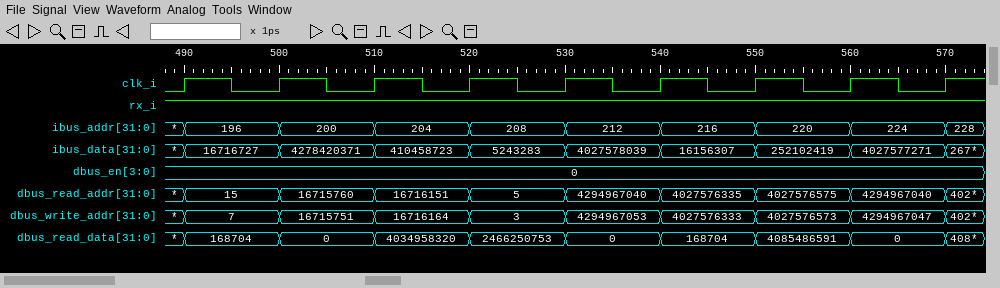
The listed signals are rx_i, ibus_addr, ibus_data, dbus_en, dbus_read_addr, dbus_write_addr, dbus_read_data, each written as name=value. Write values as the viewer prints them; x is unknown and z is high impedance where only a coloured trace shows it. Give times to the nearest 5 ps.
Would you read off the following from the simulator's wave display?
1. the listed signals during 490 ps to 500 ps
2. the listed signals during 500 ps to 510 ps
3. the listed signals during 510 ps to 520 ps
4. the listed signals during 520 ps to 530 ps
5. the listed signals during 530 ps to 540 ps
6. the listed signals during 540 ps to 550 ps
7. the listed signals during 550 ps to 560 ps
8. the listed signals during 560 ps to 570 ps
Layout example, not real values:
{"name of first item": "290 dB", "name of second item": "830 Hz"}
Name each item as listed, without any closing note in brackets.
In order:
{"the listed signals during 490 ps to 500 ps": "rx_i=1, ibus_addr=196, ibus_data=16716727, dbus_en=0, dbus_read_addr=15, dbus_write_addr=7, dbus_read_data=168704", "the listed signals during 500 ps to 510 ps": "rx_i=1, ibus_addr=200, ibus_data=4278420371, dbus_en=0, dbus_read_addr=16715760, dbus_write_addr=16715751, dbus_read_data=0", "the listed signals during 510 ps to 520 ps": "rx_i=1, ibus_addr=204, ibus_data=410458723, dbus_en=0, dbus_read_addr=16716151, dbus_write_addr=16716164, dbus_read_data=4034958320", "the listed signals during 520 ps to 530 ps": "rx_i=1, ibus_addr=208, ibus_data=5243283, dbus_en=0, dbus_read_addr=5, dbus_write_addr=3, dbus_read_data=2466250753", "the listed signals during 530 ps to 540 ps": "rx_i=1, ibus_addr=212, ibus_data=4027578039, dbus_en=0, dbus_read_addr=4294967040, dbus_write_addr=4294967053, dbus_read_data=0", "the listed signals during 540 ps to 550 ps": "rx_i=1, ibus_addr=216, ibus_data=16156307, dbus_en=0, dbus_read_addr=4027576335, dbus_write_addr=4027576333, dbus_read_data=168704", "the listed signals during 550 ps to 560 ps": "rx_i=1, ibus_addr=220, ibus_data=252102419, dbus_en=0, dbus_read_addr=4027576575, dbus_write_addr=4027576573, dbus_read_data=4085486591", "the listed signals during 560 ps to 570 ps": "rx_i=1, ibus_addr=224, ibus_data=4027577271, dbus_en=0, dbus_read_addr=4294967040, dbus_write_addr=4294967047, dbus_read_data=0"}
